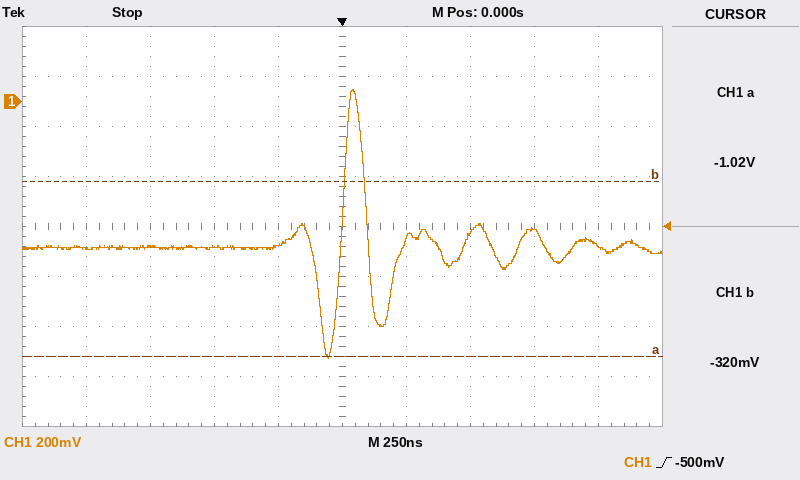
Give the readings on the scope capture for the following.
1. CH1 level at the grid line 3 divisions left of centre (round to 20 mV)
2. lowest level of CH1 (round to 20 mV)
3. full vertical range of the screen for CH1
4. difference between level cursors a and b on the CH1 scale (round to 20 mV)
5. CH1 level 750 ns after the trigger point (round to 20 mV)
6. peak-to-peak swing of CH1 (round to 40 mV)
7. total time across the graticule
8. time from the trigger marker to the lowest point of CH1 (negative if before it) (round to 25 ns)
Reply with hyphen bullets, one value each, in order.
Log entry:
- -580 mV
- -1.02 V
- 1.6 V
- 700 mV
- -520 mV
- 1.08 V
- 2.5 µs
- -50 ns
